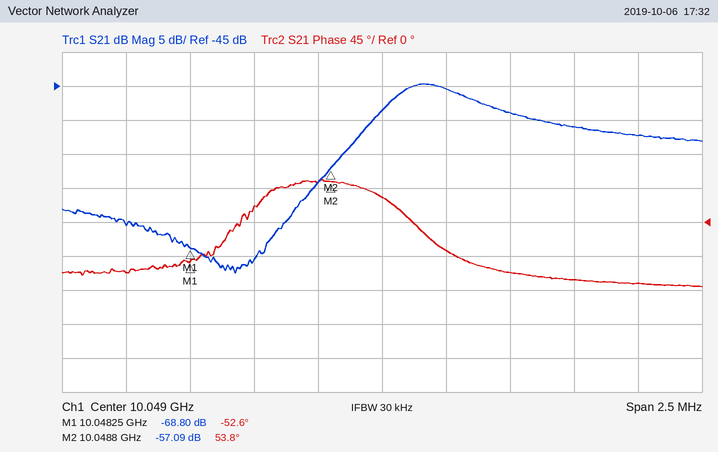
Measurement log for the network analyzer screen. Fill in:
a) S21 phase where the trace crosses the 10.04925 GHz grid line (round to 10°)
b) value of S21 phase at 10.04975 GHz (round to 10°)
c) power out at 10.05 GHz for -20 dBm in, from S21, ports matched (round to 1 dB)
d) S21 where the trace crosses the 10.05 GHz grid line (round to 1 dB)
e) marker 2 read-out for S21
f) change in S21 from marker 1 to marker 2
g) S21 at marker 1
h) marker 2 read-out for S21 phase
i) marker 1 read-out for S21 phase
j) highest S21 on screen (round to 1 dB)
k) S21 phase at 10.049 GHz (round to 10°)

-40°
-80°
-72 dBm
-52 dB
-57.09 dB
11.71 dB
-68.80 dB
53.8°
-52.6°
-45 dB
30°
